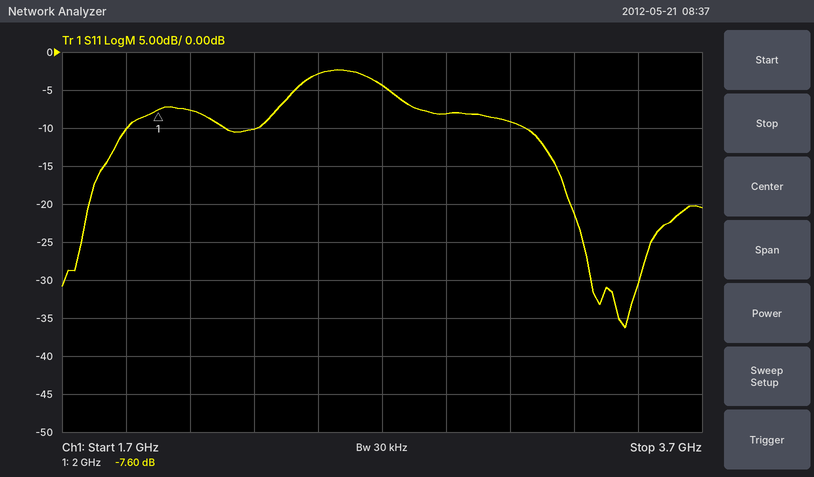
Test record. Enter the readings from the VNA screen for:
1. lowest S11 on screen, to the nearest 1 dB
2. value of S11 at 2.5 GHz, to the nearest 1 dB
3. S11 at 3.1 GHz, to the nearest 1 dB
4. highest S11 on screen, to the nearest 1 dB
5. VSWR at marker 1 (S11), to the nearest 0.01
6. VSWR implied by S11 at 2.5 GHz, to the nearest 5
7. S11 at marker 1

-36 dB
-3 dB
-9 dB
-2 dB
2.43
5
-7.60 dB
